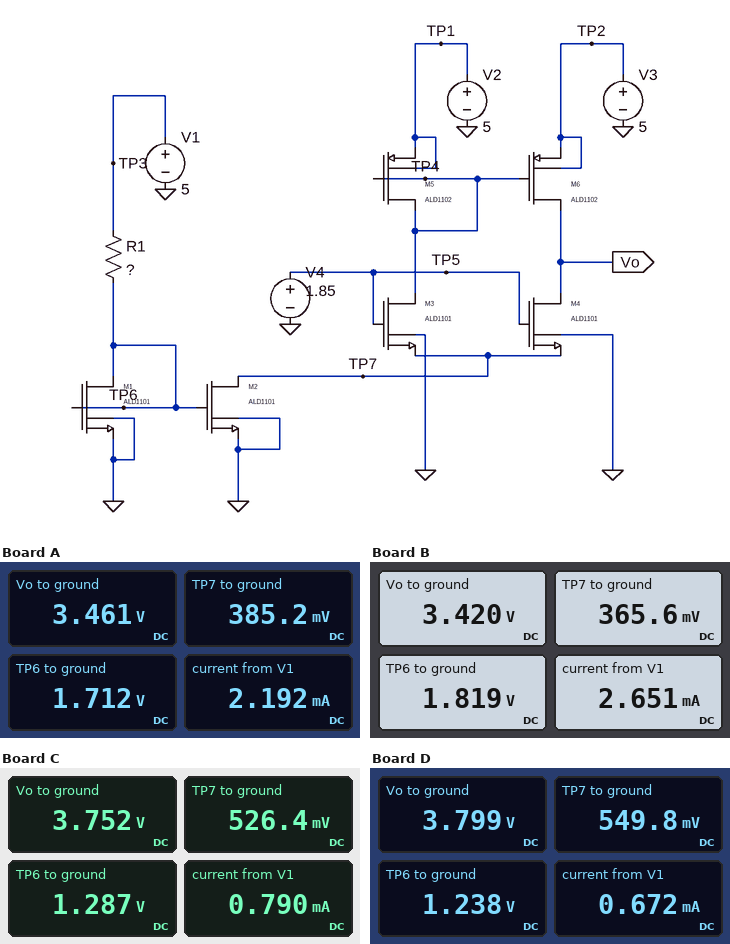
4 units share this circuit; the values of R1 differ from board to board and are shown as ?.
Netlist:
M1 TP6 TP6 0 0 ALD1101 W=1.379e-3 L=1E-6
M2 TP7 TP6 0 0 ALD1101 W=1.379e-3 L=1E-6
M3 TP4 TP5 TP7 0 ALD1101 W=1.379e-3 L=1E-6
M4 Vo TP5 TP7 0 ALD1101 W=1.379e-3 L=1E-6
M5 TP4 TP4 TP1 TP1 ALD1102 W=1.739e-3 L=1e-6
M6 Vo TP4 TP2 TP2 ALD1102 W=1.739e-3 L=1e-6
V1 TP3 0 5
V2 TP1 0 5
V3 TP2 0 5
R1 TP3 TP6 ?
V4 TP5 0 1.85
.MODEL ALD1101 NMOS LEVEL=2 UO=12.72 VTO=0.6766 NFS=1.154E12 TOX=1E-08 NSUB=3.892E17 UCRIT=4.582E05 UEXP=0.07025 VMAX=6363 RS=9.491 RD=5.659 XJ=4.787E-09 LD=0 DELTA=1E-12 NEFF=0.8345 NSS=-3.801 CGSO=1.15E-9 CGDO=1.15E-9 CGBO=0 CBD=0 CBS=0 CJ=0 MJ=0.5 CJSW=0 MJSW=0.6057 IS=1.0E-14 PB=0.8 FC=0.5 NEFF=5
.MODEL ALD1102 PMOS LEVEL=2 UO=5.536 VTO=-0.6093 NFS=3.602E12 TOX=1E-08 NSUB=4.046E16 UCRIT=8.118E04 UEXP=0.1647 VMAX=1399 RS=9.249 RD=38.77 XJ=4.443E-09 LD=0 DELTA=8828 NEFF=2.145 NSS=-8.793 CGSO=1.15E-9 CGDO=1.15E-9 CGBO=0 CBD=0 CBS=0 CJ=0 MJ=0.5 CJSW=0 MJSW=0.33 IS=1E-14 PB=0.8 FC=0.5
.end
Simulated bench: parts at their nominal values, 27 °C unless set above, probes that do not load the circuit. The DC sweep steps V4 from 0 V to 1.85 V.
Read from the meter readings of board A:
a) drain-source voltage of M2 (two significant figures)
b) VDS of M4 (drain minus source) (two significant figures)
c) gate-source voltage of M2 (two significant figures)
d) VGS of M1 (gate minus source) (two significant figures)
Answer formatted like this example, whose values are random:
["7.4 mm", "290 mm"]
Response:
["390 mV", "3.1 V", "1.7 V", "1.7 V"]
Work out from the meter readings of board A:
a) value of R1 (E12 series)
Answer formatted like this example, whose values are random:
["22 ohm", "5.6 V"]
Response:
["1.5 kΩ"]
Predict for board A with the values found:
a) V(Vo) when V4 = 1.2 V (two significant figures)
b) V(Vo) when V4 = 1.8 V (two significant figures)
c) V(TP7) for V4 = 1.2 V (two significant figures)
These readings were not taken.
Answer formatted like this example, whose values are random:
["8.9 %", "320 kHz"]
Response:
["3.8 V", "3.5 V", "110 mV"]
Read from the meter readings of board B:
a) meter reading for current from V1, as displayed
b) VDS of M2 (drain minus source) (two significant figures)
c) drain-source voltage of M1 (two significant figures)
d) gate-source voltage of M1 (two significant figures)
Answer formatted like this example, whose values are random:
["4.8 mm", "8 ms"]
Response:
["2.651 mA", "370 mV", "1.8 V", "1.8 V"]
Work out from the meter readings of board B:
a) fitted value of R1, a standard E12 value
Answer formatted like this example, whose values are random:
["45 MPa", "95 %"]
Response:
["1.2 kΩ"]
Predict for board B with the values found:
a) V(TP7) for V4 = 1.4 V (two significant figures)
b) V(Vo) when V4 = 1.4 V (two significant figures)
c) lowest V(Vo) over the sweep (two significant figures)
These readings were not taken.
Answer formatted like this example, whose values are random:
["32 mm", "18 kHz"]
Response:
["170 mV", "3.7 V", "3.4 V"]
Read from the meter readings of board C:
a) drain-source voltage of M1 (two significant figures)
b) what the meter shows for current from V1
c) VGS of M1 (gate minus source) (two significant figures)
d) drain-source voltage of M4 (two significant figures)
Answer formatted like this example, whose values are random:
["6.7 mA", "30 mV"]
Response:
["1.3 V", "0.790 mA", "1.3 V", "3.2 V"]
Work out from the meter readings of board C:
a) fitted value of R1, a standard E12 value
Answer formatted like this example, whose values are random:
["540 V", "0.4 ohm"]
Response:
["4.7 kΩ"]
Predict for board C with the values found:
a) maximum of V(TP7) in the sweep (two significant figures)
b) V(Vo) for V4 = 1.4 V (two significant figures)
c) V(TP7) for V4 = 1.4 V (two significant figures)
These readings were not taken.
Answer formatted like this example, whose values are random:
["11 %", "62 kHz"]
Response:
["530 mV", "3.8 V", "240 mV"]
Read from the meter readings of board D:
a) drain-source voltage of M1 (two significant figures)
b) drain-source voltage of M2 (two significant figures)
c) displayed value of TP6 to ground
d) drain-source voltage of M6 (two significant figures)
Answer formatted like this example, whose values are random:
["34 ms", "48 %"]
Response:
["1.2 V", "550 mV", "1.238 V", "-1.2 V"]
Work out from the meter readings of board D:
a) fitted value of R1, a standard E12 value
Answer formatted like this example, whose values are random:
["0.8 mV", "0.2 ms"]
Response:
["5.6 kΩ"]
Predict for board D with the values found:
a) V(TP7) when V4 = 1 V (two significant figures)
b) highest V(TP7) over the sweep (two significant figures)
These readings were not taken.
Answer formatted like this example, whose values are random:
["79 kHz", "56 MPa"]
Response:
["75 mV", "550 mV"]
